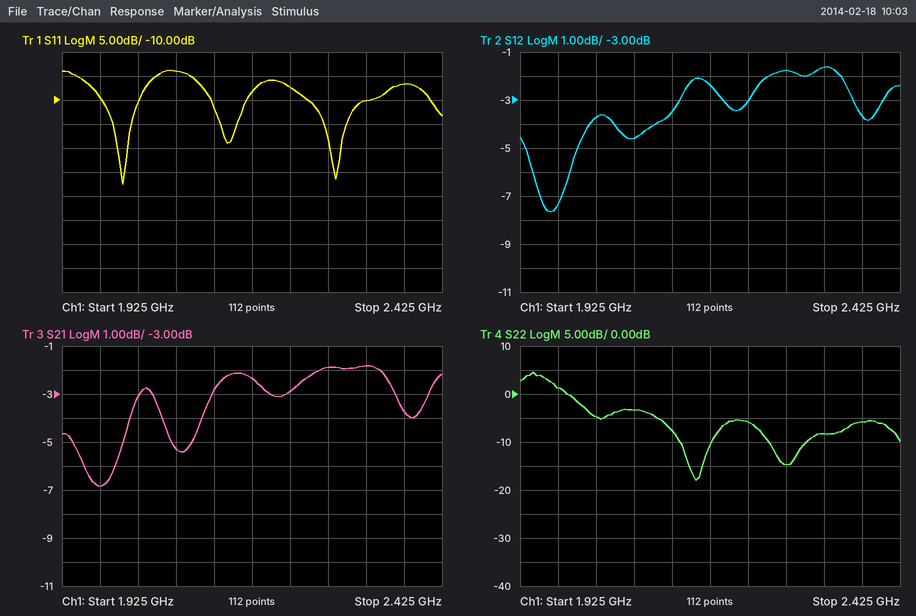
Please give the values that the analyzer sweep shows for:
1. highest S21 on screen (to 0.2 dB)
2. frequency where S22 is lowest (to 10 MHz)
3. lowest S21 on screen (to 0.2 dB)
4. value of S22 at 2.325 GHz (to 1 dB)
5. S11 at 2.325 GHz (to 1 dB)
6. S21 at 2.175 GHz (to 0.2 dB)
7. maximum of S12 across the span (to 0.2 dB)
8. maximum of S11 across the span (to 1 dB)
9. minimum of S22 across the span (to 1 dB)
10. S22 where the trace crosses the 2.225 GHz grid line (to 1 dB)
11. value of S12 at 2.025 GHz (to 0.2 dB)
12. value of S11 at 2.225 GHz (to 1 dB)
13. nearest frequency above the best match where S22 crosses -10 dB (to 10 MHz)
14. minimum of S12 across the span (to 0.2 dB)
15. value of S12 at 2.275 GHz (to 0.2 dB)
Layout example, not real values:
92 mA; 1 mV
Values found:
-1.8 dB; 2.16 GHz; -6.8 dB; -8 dB; -10 dB; -2.4 dB; -1.6 dB; -4 dB; -18 dB; -6 dB; -3.8 dB; -7 dB; 2.18 GHz; -7.6 dB; -1.8 dB
